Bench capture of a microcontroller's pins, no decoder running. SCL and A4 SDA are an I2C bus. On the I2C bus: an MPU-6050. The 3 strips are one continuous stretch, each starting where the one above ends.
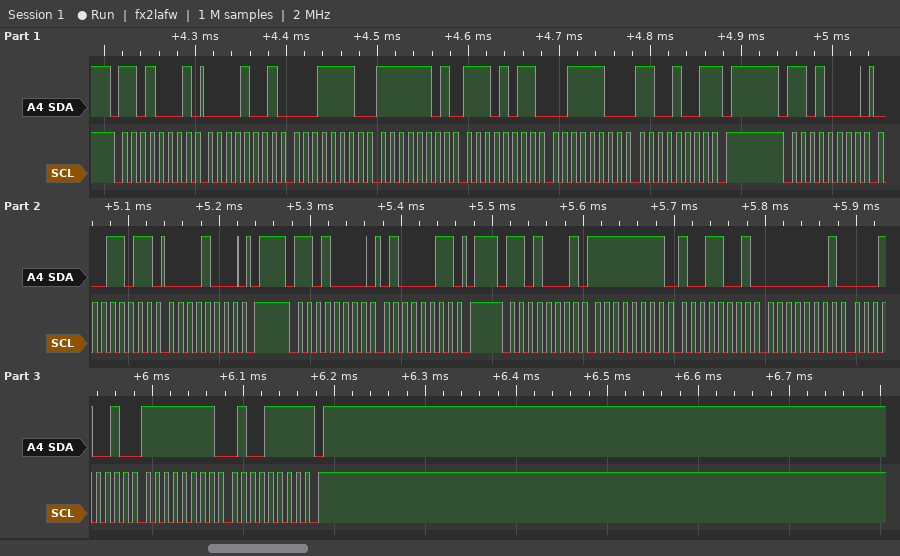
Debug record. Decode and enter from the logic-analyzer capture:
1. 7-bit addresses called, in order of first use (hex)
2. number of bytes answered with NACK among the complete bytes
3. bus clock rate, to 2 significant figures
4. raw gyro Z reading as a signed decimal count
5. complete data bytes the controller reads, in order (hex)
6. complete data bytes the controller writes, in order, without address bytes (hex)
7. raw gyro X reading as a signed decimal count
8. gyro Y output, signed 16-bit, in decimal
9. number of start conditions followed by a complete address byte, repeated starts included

0x68
2
100 kHz
-177
09 1E FD EB 3C C9 FF 99 01 12 FF 4F
1B 08 43
-103
274
4
